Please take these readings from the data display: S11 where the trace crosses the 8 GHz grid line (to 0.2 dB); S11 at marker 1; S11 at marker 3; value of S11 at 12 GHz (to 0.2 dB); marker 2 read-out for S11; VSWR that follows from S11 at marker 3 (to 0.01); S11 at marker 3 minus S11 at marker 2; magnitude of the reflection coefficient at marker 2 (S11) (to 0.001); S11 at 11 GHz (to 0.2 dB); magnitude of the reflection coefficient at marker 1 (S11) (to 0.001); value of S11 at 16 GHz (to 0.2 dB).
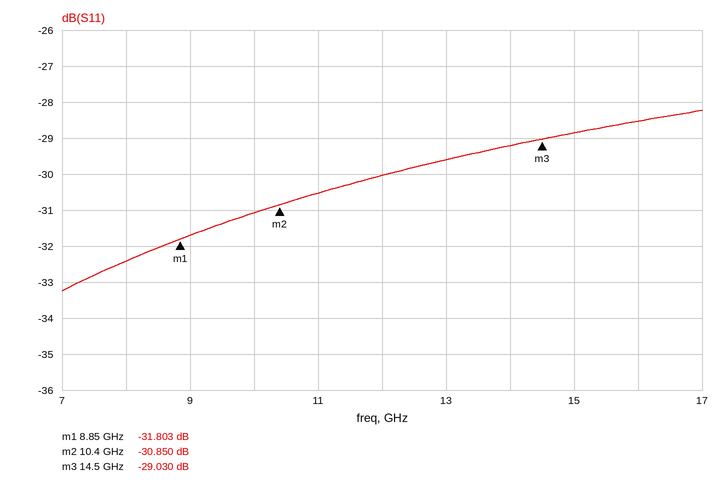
-32.4 dB
-31.803 dB
-29.030 dB
-30.0 dB
-30.850 dB
1.07
1.820 dB
0.029
-30.6 dB
0.026
-28.6 dB
